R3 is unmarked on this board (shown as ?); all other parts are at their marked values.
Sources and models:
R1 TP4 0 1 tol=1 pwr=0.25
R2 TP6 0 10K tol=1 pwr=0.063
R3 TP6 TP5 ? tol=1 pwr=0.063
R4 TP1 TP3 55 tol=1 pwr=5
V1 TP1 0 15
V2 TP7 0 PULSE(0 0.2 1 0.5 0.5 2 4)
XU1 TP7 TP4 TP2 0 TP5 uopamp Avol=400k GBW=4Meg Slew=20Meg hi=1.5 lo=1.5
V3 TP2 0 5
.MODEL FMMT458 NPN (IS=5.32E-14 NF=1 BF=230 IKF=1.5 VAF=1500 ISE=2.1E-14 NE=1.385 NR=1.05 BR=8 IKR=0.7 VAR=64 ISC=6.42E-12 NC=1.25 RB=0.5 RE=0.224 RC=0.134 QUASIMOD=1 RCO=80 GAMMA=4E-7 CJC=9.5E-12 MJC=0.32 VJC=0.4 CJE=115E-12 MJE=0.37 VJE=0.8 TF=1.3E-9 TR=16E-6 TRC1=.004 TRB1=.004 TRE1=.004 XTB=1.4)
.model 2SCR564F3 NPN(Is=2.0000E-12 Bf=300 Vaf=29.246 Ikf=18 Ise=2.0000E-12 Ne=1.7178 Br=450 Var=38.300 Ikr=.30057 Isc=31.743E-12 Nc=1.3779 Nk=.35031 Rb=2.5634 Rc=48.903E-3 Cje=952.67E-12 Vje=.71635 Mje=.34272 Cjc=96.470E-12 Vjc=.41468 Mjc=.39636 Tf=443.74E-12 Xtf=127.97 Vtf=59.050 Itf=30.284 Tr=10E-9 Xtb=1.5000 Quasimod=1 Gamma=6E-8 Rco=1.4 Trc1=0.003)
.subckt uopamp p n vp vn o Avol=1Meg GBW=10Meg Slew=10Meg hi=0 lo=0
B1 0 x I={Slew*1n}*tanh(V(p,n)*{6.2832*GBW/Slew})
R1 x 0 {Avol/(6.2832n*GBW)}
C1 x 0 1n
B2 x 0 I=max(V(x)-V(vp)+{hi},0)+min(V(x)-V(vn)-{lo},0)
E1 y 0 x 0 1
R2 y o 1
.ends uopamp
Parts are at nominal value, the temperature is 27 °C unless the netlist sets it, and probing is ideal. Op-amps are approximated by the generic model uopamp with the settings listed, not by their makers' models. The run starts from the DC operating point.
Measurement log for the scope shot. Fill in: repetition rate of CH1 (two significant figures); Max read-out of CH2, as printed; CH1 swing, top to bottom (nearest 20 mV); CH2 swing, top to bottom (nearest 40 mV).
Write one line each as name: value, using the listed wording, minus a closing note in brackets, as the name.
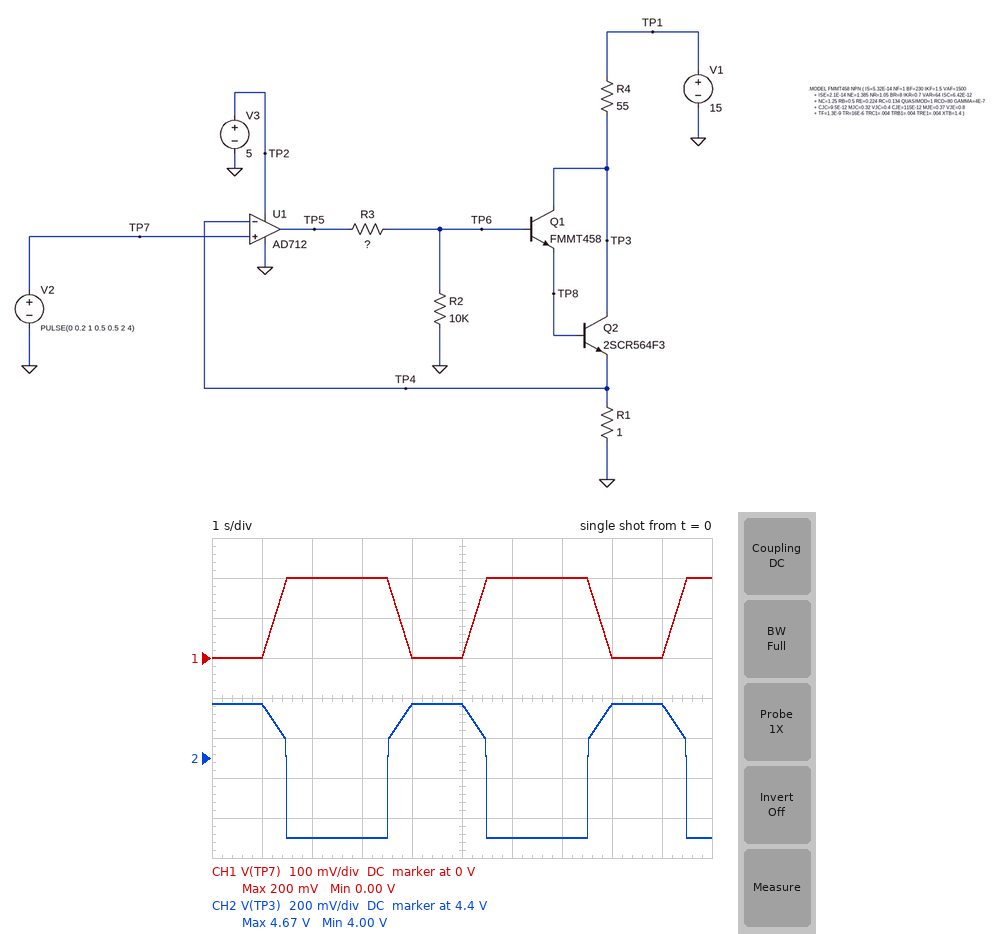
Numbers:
repetition rate of CH1: 250 mHz
Max read-out of CH2, as printed: 4.67 V
CH1 swing, top to bottom: 200 mV
CH2 swing, top to bottom: 680 mV
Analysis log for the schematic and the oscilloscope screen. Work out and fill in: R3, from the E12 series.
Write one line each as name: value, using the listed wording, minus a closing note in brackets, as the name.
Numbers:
R3, from the E12 series: 390 Ω
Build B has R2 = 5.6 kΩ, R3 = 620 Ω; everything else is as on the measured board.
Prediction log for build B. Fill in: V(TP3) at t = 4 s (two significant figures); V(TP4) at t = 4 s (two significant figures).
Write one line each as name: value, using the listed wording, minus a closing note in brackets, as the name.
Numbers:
V(TP3) at t = 4 s: 8.2 V
V(TP4) at t = 4 s: 120 mV
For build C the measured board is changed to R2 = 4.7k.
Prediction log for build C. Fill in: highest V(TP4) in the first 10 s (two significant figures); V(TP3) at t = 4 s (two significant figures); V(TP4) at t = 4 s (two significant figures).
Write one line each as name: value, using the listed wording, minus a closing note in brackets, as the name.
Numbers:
highest V(TP4) in the first 10 s: 200 mV
V(TP3) at t = 4 s: 6.9 V
V(TP4) at t = 4 s: 150 mV
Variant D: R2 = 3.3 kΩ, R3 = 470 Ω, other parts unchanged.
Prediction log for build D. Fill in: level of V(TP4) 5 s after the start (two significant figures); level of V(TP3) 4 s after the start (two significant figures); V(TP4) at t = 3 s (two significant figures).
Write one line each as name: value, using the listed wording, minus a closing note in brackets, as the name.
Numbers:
level of V(TP4) 5 s after the start: 100 mV
level of V(TP3) 4 s after the start: 9.5 V
V(TP4) at t = 3 s: 200 mV
